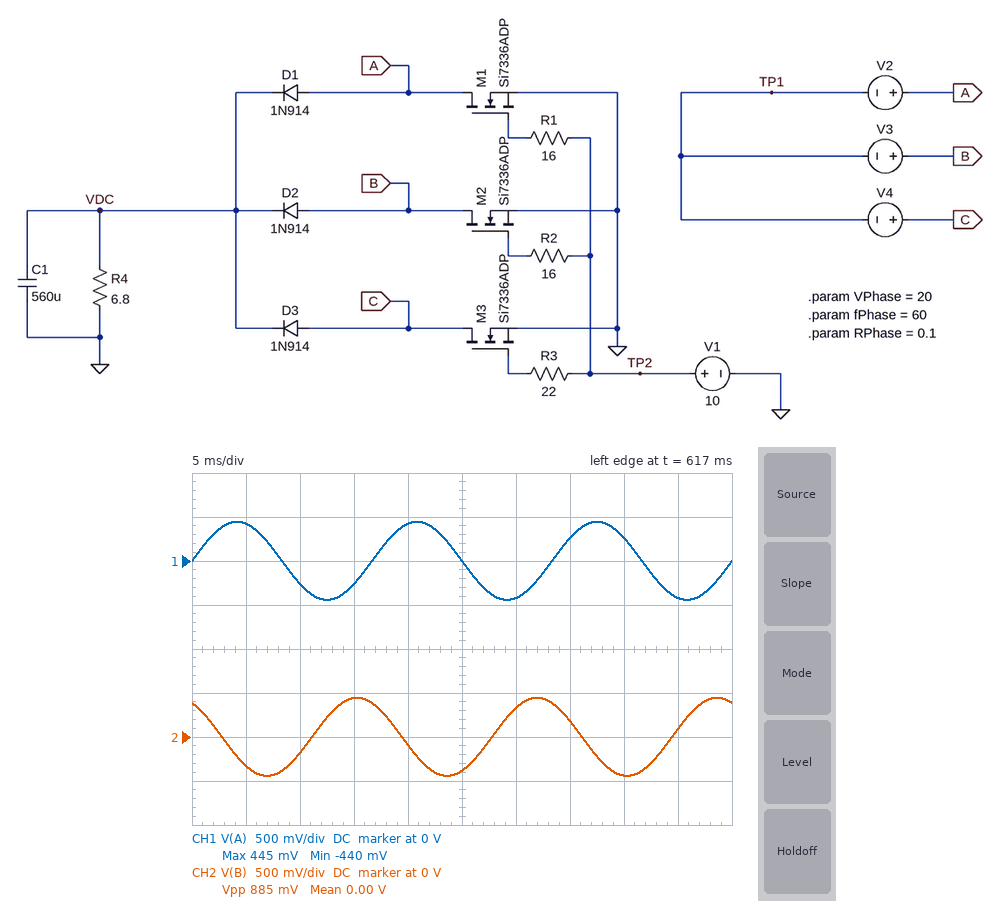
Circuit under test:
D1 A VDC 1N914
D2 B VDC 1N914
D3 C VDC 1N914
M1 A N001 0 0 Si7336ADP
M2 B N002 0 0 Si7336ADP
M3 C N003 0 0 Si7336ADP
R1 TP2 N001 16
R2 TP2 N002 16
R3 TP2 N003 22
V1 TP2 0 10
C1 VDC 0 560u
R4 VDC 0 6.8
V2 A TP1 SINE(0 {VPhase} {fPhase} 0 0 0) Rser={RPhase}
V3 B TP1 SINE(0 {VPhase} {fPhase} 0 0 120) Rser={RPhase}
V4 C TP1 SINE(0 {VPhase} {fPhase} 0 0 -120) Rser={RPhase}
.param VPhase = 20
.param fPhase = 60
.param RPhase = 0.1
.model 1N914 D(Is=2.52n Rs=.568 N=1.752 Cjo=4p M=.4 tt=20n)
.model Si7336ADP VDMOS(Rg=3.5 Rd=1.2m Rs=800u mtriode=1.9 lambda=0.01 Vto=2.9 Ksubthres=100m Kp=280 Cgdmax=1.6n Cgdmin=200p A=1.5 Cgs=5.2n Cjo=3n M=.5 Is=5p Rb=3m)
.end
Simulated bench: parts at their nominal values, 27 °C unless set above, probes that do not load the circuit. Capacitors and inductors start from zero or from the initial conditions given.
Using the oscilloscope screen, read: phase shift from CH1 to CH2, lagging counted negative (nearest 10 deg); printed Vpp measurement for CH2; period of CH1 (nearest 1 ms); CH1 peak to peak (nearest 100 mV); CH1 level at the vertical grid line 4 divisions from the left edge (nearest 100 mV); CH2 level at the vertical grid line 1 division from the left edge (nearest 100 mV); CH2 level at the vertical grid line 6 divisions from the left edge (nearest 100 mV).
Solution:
120 deg
885 mV
17 ms
900 mV
400 mV
-300 mV
300 mV
